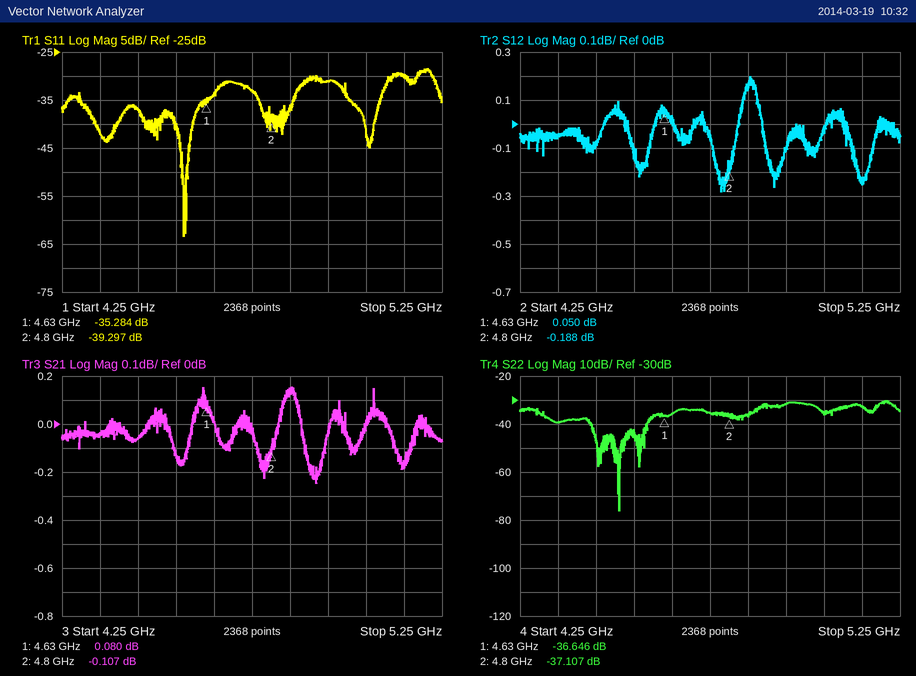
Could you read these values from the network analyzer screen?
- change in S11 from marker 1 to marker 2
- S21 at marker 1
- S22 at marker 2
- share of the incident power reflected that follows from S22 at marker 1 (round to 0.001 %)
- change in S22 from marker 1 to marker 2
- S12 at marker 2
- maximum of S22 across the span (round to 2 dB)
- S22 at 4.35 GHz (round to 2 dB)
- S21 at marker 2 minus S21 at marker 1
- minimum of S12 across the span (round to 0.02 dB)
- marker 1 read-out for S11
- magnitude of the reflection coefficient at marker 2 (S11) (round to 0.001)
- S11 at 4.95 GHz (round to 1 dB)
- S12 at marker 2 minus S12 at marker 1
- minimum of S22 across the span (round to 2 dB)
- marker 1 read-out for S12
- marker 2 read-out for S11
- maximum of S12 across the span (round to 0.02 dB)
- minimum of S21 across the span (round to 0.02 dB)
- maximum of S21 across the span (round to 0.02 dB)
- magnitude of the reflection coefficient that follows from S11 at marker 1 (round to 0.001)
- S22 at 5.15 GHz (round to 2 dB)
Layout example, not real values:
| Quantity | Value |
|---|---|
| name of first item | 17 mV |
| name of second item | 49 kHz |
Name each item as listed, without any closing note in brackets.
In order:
| Quantity | Value |
|---|---|
| change in S11 from marker 1 to marker 2 | -4.013 dB |
| S21 at marker 1 | 0.080 dB |
| S22 at marker 2 | -37.107 dB |
| share of the incident power reflected that follows from S22 at marker 1 | 0.022 % |
| change in S22 from marker 1 to marker 2 | -0.461 dB |
| S12 at marker 2 | -0.188 dB |
| maximum of S22 across the span | -30 dB |
| S22 at 4.35 GHz | -40 dB |
| S21 at marker 2 minus S21 at marker 1 | -0.187 dB |
| minimum of S12 across the span | -0.28 dB |
| marker 1 read-out for S11 | -35.284 dB |
| magnitude of the reflection coefficient at marker 2 (S11) | 0.011 |
| S11 at 4.95 GHz | -31 dB |
| S12 at marker 2 minus S12 at marker 1 | -0.238 dB |
| minimum of S22 across the span | -76 dB |
| marker 1 read-out for S12 | 0.050 dB |
| marker 2 read-out for S11 | -39.297 dB |
| maximum of S12 across the span | 0.20 dB |
| minimum of S21 across the span | -0.24 dB |
| maximum of S21 across the span | 0.16 dB |
| magnitude of the reflection coefficient that follows from S11 at marker 1 | 0.017 |
| S22 at 5.15 GHz | -32 dB |
